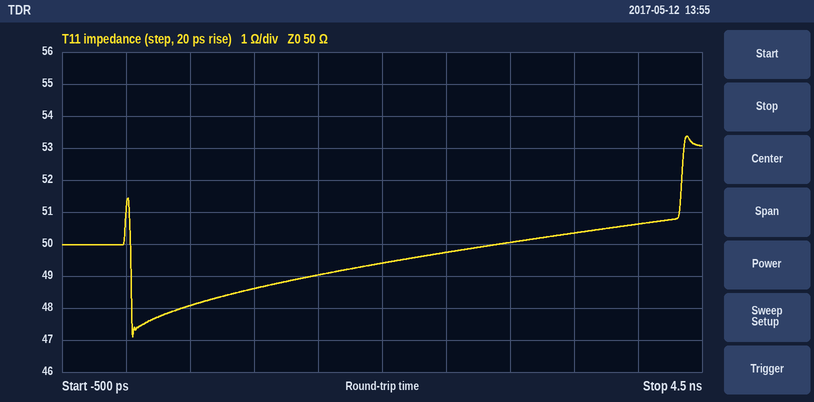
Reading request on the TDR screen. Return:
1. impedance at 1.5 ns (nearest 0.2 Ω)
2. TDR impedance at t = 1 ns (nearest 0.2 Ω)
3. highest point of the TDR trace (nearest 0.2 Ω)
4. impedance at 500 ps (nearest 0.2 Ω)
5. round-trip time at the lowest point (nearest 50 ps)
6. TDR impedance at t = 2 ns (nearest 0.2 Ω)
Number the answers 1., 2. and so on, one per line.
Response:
1. 49.0 Ω
2. 48.6 Ω
3. 53.4 Ω
4. 48.0 Ω
5. 50 ps
6. 49.4 Ω
